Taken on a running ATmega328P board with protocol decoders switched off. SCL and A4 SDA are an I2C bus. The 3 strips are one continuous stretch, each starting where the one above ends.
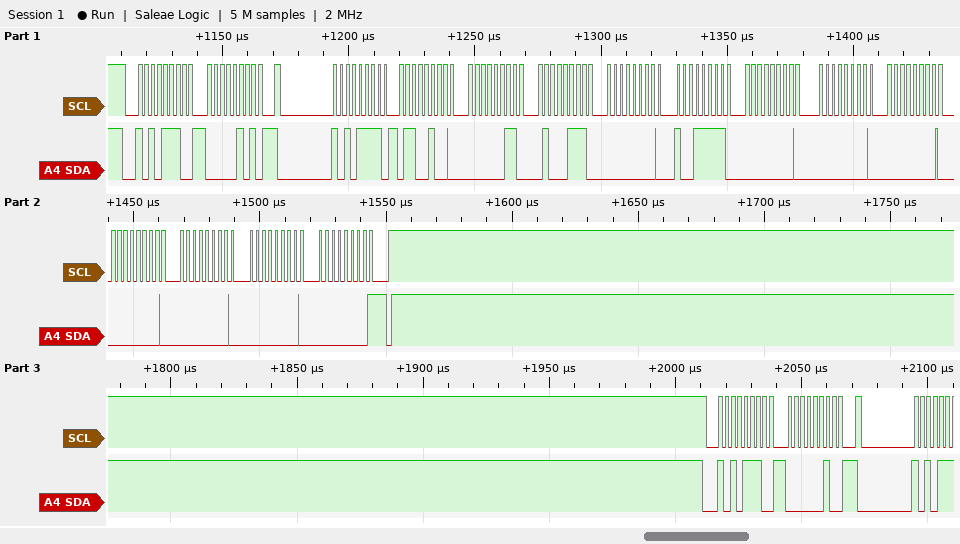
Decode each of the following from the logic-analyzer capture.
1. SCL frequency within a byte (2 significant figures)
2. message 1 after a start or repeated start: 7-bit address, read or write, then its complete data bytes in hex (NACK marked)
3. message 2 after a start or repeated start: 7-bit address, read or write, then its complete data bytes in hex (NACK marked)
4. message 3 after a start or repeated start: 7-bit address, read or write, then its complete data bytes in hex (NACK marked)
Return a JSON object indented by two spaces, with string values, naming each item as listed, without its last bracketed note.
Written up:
{
  "SCL frequency within a byte": "400 kHz",
  "message 1 after a start or repeated start: 7-bit address, read or write, then its complete data bytes in hex": "0x57 write: 05",
  "message 2 after a start or repeated start: 7-bit address, read or write, then its complete data bytes in hex": "0x57 read: 64 03 47 00 9F 00 00 00 00 00 00 00 NACK",
  "message 3 after a start or repeated start: 7-bit address, read or write, then its complete data bytes in hex": "0x57 write: 02"
}
